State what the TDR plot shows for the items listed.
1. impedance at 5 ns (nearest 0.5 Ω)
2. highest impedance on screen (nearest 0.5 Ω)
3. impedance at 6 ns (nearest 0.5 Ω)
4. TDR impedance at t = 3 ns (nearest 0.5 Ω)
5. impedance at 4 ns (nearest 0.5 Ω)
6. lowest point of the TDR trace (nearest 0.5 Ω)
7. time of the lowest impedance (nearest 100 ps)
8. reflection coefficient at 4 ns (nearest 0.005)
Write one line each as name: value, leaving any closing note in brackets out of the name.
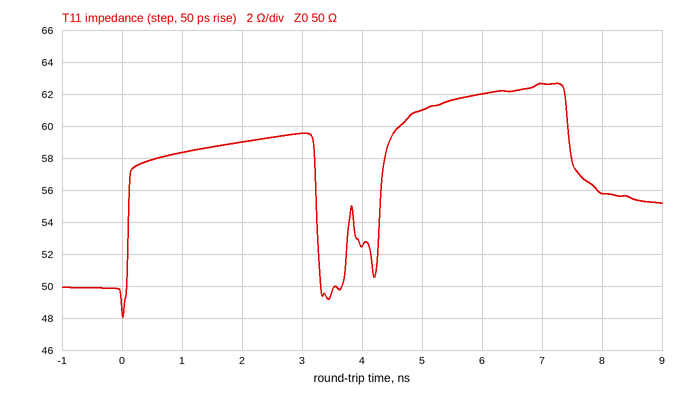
impedance at 5 ns: 61.0 Ω
highest impedance on screen: 62.5 Ω
impedance at 6 ns: 62.0 Ω
TDR impedance at t = 3 ns: 59.5 Ω
impedance at 4 ns: 52.5 Ω
lowest point of the TDR trace: 48.0 Ω
time of the lowest impedance: 0.0 ns
reflection coefficient at 4 ns: +0.025
